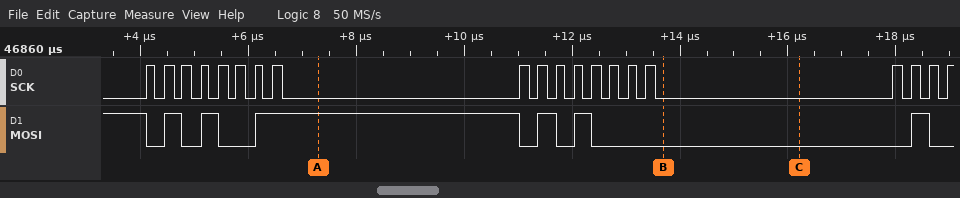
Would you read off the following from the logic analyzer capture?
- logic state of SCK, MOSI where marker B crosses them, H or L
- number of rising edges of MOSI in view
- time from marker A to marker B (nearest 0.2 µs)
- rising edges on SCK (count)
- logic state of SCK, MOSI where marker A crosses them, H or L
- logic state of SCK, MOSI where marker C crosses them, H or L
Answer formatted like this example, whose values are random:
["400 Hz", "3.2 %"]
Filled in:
["SCK=L, MOSI=L", "6", "6.4 µs", "20", "SCK=L, MOSI=H", "SCK=L, MOSI=L"]
